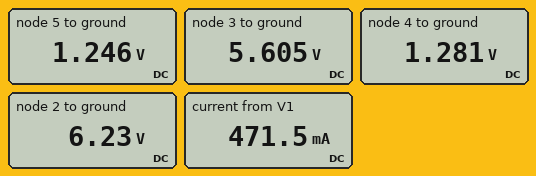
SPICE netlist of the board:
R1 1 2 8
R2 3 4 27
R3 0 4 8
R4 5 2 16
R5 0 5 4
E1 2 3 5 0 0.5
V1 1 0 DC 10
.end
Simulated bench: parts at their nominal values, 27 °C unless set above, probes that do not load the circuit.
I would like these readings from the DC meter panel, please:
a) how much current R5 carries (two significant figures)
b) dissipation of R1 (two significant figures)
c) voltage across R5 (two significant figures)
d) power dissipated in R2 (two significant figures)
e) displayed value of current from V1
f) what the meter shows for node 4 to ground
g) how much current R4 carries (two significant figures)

310 mA
1.8 W
1.2 V
690 mW
471.5 mA
1.281 V
310 mA
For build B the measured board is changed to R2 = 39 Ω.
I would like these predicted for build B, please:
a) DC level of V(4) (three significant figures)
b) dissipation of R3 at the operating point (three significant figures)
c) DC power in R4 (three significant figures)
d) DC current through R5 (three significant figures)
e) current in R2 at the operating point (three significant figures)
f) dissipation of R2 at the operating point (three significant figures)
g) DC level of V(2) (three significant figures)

986 mV
122 mW
1.66 W
322 mA
123 mA
593 mW
6.44 V
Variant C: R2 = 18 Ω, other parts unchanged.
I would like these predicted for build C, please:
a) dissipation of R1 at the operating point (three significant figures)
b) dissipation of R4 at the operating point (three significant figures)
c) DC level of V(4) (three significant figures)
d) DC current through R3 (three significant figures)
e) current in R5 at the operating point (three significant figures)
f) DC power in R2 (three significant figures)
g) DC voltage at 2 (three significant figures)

2.04 W
1.42 W
1.65 V
206 mA
298 mA
767 mW
5.96 V
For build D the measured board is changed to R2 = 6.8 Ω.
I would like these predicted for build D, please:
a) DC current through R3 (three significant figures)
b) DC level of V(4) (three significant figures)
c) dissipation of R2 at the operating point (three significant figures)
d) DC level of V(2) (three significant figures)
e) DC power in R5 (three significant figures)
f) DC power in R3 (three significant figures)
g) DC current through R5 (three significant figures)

322 mA
2.58 V
707 mW
5.30 V
281 mW
831 mW
265 mA
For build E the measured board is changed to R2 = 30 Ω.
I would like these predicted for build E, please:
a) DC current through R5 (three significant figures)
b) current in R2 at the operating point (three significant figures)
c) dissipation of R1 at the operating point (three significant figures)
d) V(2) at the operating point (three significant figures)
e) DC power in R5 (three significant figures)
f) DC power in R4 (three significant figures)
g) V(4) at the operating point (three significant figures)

315 mA
149 mA
1.72 W
6.29 V
396 mW
1.58 W
1.19 V
